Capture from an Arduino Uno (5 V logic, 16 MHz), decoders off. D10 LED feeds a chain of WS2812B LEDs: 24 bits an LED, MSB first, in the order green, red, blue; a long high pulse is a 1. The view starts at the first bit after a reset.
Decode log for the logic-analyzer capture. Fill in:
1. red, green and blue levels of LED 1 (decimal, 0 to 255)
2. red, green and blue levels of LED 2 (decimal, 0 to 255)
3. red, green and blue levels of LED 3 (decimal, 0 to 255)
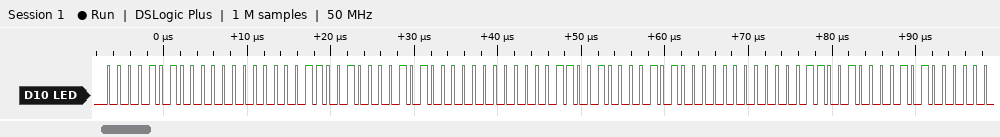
0, 10, 25
0, 10, 25
0, 10, 25
